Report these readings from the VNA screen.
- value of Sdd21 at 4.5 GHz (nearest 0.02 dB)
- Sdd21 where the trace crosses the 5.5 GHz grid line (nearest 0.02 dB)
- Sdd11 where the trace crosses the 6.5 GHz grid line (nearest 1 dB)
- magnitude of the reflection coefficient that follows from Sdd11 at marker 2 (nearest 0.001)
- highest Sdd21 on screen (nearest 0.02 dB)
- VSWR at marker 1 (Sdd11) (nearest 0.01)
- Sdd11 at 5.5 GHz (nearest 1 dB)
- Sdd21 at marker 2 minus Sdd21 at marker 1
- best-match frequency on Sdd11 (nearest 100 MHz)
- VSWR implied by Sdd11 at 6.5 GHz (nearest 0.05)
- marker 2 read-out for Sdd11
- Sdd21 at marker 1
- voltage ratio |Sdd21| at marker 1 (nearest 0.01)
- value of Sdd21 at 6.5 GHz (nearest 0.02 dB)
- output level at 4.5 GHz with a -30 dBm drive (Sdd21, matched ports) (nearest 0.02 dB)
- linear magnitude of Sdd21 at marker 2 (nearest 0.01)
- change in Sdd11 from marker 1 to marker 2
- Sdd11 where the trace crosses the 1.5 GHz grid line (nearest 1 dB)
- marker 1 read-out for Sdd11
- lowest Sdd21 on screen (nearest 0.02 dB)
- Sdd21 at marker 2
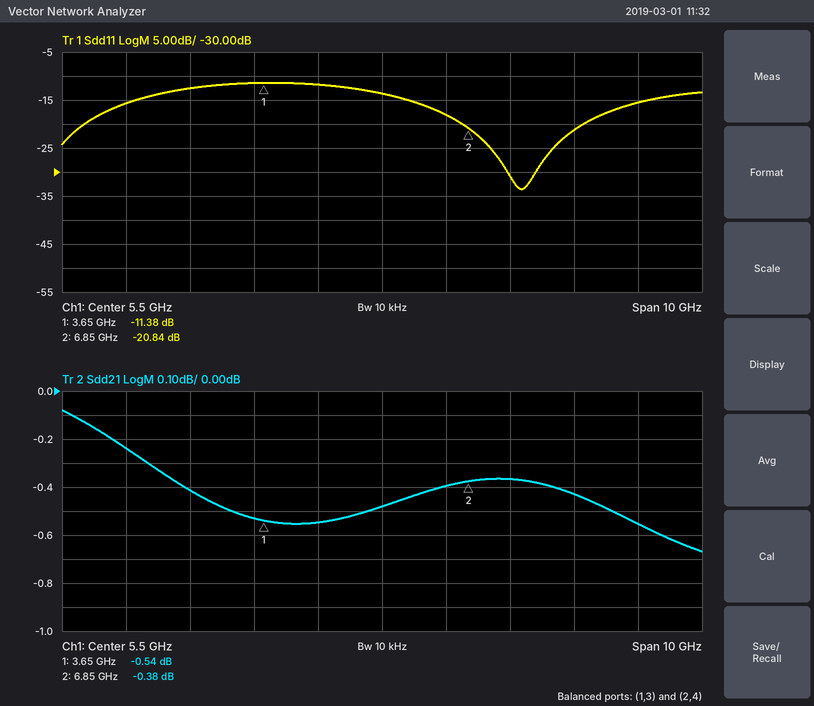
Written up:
-0.54 dB
-0.48 dB
-18 dB
0.091
-0.08 dB
1.74
-14 dB
0.16 dB
7.7 GHz
1.30
-20.84 dB
-0.54 dB
0.94
-0.40 dB
-30.54 dBm
0.96
-9.46 dB
-16 dB
-11.38 dB
-0.66 dB
-0.38 dB
